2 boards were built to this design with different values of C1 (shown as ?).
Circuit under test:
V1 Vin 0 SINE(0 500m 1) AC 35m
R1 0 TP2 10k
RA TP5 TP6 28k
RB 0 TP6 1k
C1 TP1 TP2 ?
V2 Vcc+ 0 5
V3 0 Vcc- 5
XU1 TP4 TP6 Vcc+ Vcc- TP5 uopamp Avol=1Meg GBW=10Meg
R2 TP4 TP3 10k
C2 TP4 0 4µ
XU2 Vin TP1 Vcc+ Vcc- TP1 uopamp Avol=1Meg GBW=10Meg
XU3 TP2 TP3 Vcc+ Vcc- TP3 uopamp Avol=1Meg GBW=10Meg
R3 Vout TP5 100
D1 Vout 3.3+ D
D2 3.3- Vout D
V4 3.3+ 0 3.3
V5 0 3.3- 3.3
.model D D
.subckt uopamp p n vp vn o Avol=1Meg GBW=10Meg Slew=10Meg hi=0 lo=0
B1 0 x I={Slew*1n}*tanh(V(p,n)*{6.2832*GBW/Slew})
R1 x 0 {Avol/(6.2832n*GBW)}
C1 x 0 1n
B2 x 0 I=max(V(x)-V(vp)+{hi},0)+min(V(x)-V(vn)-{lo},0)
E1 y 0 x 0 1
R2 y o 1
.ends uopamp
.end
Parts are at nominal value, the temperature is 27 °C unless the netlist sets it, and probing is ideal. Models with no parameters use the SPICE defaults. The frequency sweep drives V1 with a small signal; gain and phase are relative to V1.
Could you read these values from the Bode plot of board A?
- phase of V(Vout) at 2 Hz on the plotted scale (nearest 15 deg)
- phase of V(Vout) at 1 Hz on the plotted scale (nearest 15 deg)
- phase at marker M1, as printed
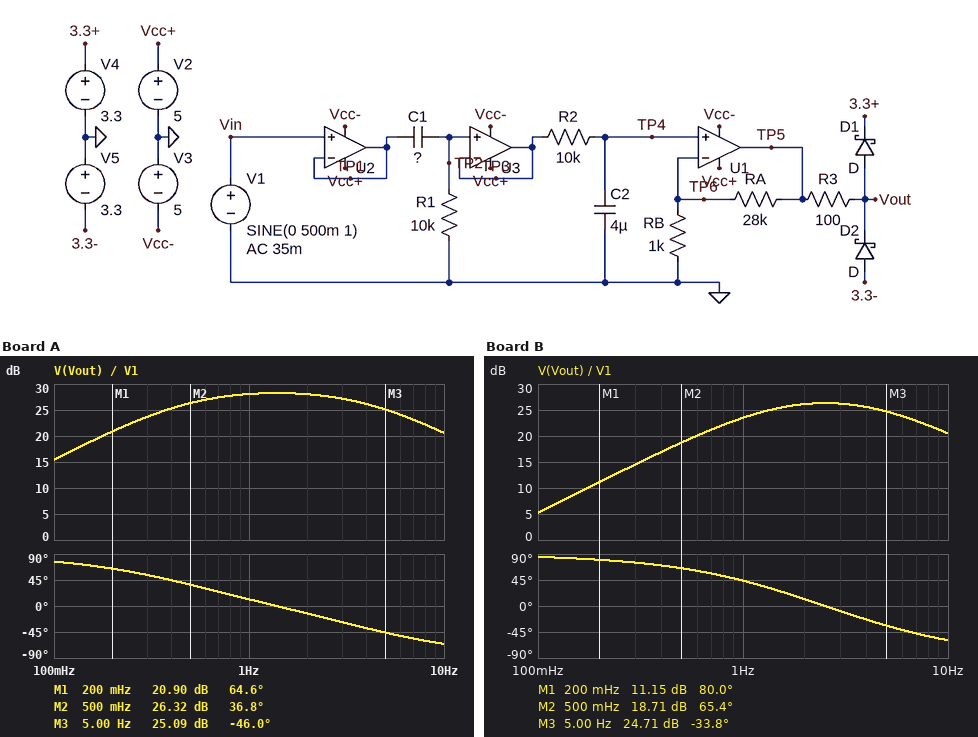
-15 deg
15 deg
64.6 deg
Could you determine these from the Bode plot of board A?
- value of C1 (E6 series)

33 µF
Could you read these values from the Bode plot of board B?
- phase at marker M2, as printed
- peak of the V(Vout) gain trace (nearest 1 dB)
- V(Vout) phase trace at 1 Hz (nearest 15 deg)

65.4 deg
26 dB
45 deg
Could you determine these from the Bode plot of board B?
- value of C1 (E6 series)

10 µF
